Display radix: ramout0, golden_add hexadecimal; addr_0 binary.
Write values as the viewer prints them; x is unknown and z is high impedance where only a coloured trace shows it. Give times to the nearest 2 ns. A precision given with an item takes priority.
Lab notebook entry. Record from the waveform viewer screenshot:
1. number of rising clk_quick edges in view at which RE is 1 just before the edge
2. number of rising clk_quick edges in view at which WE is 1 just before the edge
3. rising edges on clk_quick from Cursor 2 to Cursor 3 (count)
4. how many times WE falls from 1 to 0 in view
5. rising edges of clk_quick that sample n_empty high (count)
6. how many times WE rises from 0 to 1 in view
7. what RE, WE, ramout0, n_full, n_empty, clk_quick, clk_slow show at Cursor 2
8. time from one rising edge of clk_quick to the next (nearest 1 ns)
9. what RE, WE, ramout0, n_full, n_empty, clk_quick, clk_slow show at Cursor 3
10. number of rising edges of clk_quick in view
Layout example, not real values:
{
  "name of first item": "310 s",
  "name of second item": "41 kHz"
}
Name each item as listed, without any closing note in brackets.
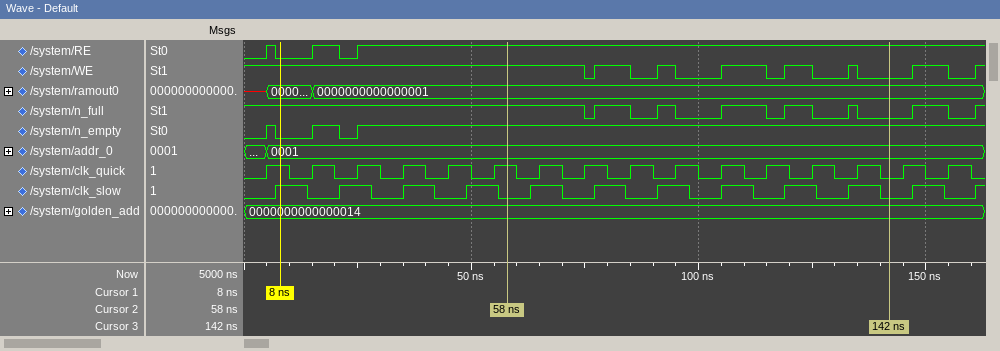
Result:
{
  "number of rising clk_quick edges in view at which RE is 1 just before the edge": "13",
  "number of rising clk_quick edges in view at which WE is 1 just before the edge": "14",
  "rising edges on clk_quick from Cursor 2 to Cursor 3": "8",
  "how many times WE falls from 1 to 0 in view": "7",
  "rising edges of clk_quick that sample n_empty high": "13",
  "how many times WE rises from 0 to 1 in view": "7",
  "what RE, WE, ramout0, n_full, n_empty, clk_quick, clk_slow show at Cursor 2": "RE=1, WE=1, ramout0=0000000000000001, n_full=1, n_empty=1, clk_quick=1, clk_slow=0",
  "time from one rising edge of clk_quick to the next": "10 ns",
  "what RE, WE, ramout0, n_full, n_empty, clk_quick, clk_slow show at Cursor 3": "RE=1, WE=0, ramout0=0000000000000001, n_full=0, n_empty=1, clk_quick=0, clk_slow=0",
  "number of rising edges of clk_quick in view": "16"
}
